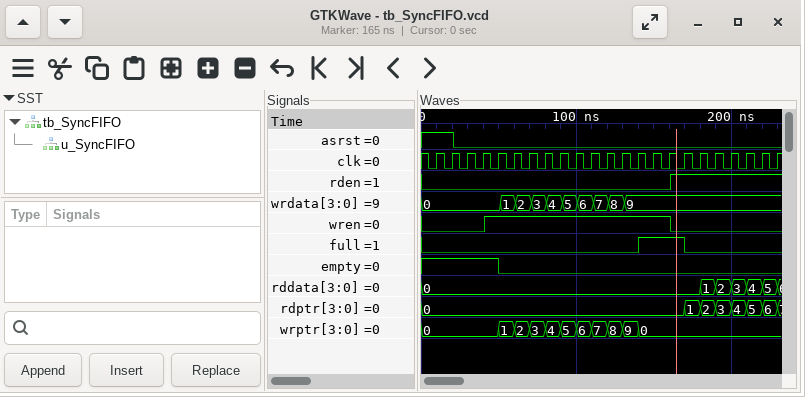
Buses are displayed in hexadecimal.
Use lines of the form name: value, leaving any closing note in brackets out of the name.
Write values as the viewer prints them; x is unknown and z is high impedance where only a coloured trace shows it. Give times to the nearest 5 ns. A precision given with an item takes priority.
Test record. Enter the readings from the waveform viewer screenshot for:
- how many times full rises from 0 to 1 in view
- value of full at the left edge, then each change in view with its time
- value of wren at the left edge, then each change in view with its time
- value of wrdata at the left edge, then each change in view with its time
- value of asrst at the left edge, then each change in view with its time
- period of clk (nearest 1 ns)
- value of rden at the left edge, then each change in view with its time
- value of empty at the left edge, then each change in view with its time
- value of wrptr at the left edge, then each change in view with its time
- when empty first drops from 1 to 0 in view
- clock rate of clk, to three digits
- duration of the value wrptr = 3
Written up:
how many times full rises from 0 to 1 in view: 1
value of full at the left edge, then each change in view with its time: 0, 1 at 140 ns, 0 at 170 ns
value of wren at the left edge, then each change in view with its time: 0, 1 at 40 ns, 0 at 160 ns
value of wrdata at the left edge, then each change in view with its time: 0, 1 at 50 ns, 2 at 60 ns, 3 at 70 ns, 4 at 80 ns, 5 at 90 ns, 6 at 100 ns, 7 at 110 ns, 8 at 120 ns, 9 at 130 ns
value of asrst at the left edge, then each change in view with its time: 1, 0 at 20 ns
period of clk: 10 ns
value of rden at the left edge, then each change in view with its time: 0, 1 at 160 ns
value of empty at the left edge, then each change in view with its time: 1, 0 at 50 ns
value of wrptr at the left edge, then each change in view with its time: 0, 1 at 50 ns, 2 at 60 ns, 3 at 70 ns, 4 at 80 ns, 5 at 90 ns, 6 at 100 ns, 7 at 110 ns, 8 at 120 ns, 9 at 130 ns, 0 at 140 ns
when empty first drops from 1 to 0 in view: 50 ns
clock rate of clk, to three digits: 100 MHz
duration of the value wrptr = 3: 10 ns
